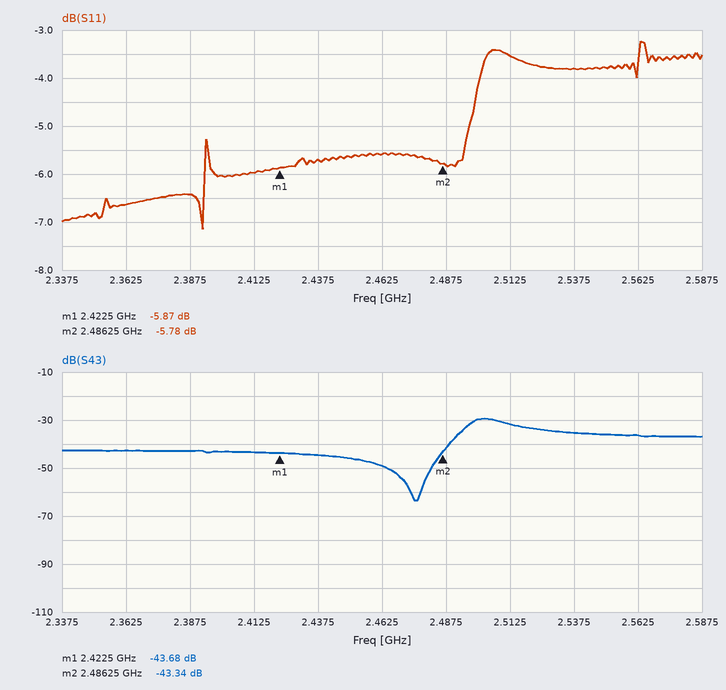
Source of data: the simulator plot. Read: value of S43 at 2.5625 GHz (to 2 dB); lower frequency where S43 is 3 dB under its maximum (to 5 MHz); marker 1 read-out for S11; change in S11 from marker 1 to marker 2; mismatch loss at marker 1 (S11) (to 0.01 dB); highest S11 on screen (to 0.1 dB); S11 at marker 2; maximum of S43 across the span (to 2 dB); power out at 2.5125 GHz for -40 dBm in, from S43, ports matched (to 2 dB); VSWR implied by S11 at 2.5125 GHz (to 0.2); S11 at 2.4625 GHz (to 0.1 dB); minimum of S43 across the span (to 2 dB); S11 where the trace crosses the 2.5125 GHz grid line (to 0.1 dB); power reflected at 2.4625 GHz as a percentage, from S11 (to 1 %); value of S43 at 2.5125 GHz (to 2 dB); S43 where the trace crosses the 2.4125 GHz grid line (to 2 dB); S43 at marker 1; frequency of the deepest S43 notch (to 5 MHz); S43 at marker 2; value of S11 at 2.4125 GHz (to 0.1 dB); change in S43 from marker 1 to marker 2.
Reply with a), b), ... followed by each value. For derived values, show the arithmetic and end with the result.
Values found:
a) -36 dB
b) 2.495 GHz
c) -5.87 dB
d) -5.78 − (-5.87) = 0.09 dB
e) −10 log10(1 − 10^(-5.87/10)) ≈ 1.30 dB
f) -3.2 dB
g) -5.78 dB
h) -30 dB
i) -40 dBm + (-32 dB) = -72 dBm
j) |Γ| = 10^(-3.5/20) = 0.6683; VSWR = (1 + 0.6683)/(1 − 0.6683) ≈ 5.0
k) -5.6 dB
l) -64 dB
m) -3.5 dB
n) 10^(-5.6/10) ≈ 28 %
o) -32 dB
p) -44 dB
q) -43.68 dB
r) 2.475 GHz
s) -43.34 dB
t) -6.0 dB
u) -43.34 − (-43.68) = 0.34 dB
